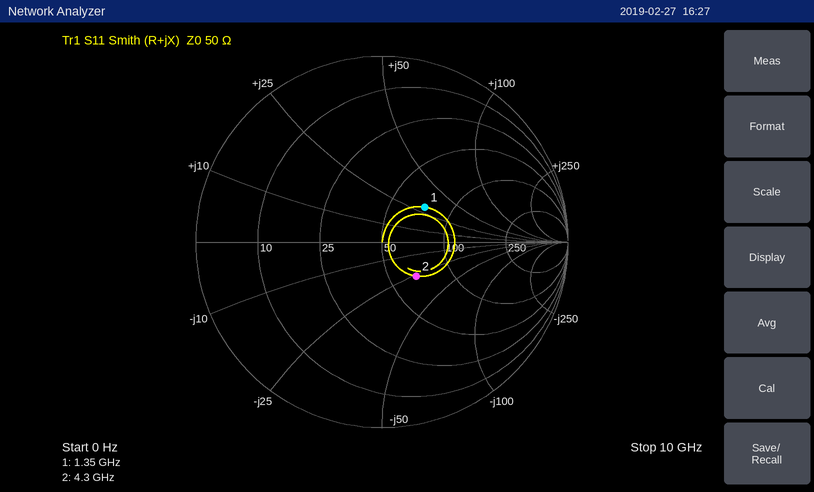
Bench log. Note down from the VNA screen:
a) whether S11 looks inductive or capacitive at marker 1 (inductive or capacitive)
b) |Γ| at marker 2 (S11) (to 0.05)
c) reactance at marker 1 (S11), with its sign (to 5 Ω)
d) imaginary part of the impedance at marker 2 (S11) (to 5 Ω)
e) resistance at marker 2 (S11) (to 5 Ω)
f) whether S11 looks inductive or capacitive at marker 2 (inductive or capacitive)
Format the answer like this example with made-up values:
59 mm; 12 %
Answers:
inductive; 0.25; +30 Ω; -25 Ω; 65 Ω; capacitive
